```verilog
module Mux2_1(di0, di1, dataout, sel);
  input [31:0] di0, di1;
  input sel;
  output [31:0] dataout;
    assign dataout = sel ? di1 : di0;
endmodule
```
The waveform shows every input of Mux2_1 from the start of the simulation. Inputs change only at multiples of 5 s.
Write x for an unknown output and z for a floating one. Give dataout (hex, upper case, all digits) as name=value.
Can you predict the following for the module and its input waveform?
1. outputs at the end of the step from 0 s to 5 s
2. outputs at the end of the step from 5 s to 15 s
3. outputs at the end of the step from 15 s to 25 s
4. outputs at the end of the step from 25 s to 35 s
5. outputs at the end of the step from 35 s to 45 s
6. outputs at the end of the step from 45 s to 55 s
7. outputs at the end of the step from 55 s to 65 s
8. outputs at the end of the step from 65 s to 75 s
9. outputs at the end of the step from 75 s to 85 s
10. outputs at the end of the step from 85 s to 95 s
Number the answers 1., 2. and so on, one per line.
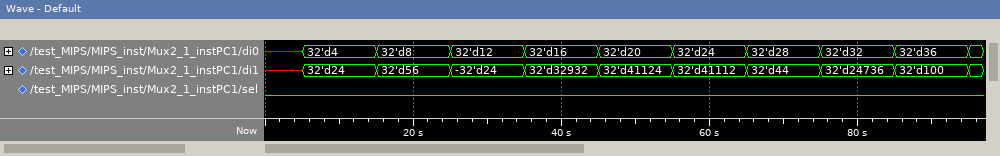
1. dataout=x
2. dataout=00000004
3. dataout=00000008
4. dataout=0000000C
5. dataout=00000010
6. dataout=00000014
7. dataout=00000018
8. dataout=0000001C
9. dataout=00000020
10. dataout=00000024
